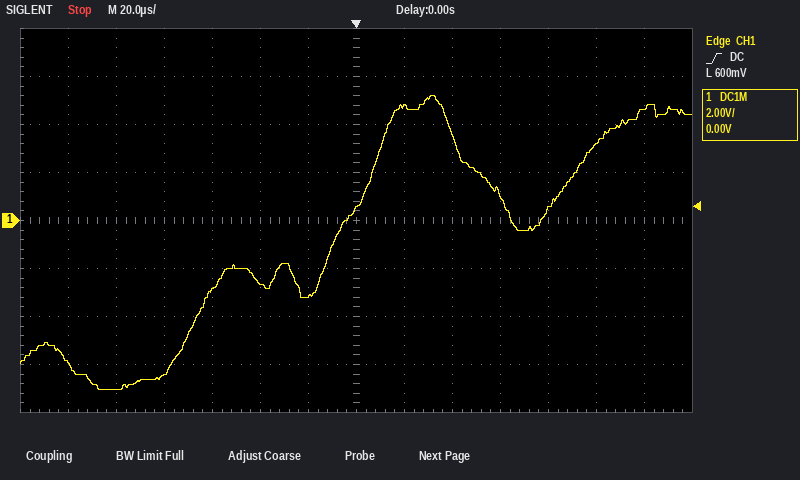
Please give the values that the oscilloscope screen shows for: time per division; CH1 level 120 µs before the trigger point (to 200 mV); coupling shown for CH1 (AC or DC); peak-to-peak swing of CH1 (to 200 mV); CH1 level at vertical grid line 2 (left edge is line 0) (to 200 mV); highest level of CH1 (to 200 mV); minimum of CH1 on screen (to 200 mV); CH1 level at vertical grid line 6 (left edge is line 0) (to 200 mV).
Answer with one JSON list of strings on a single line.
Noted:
["20 µs", "-6.0 V", "DC", "12.2 V", "-7.0 V", "5.2 V", "-7.0 V", "-3.2 V"]
